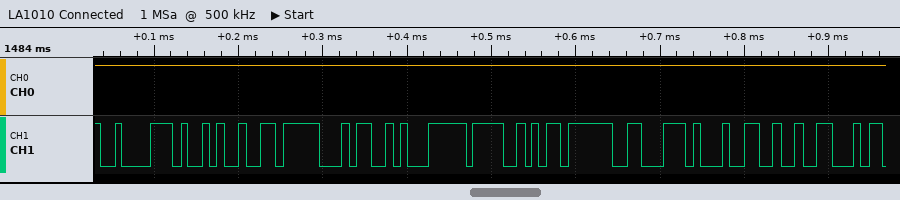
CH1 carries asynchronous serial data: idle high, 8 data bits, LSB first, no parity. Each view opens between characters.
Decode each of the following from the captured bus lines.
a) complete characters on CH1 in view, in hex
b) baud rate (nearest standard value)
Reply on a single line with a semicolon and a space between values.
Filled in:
C2, 29, F6, 34, F1, 4F, FB, C6, 91, 92; 115200 baud
